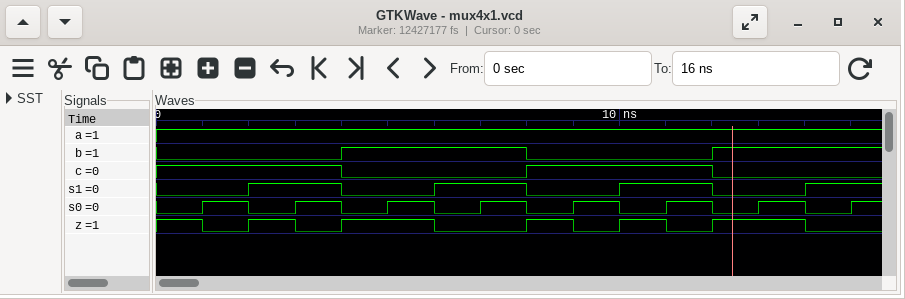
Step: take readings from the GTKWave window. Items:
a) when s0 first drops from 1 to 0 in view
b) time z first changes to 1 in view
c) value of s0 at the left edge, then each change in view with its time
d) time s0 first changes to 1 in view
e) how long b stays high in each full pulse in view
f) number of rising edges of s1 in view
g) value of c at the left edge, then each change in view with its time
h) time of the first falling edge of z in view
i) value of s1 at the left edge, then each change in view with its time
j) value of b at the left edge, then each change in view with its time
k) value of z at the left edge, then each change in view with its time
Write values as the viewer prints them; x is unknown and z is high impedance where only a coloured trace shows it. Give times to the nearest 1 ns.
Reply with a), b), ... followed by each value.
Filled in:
a) 2 ns
b) 2 ns
c) 0, 1 at 1 ns, 0 at 2 ns, 1 at 3 ns, 0 at 4 ns, 1 at 5 ns, 0 at 6 ns, 1 at 7 ns, 0 at 8 ns, 1 at 9 ns, 0 at 10 ns, 1 at 11 ns, 0 at 12 ns, 1 at 13 ns, 0 at 14 ns, 1 at 15 ns
d) 1 ns
e) 4 ns
f) 4
g) 1, 0 at 4 ns, 1 at 8 ns, 0 at 12 ns
h) 1 ns
i) 0, 1 at 2 ns, 0 at 4 ns, 1 at 6 ns, 0 at 8 ns, 1 at 10 ns, 0 at 12 ns, 1 at 14 ns
j) 0, 1 at 4 ns, 0 at 8 ns, 1 at 12 ns
k) 1, 0 at 1 ns, 1 at 2 ns, 0 at 3 ns, 1 at 4 ns, 0 at 6 ns, 1 at 8 ns, 0 at 9 ns, 1 at 10 ns, 0 at 11 ns, 1 at 12 ns, 0 at 14 ns
